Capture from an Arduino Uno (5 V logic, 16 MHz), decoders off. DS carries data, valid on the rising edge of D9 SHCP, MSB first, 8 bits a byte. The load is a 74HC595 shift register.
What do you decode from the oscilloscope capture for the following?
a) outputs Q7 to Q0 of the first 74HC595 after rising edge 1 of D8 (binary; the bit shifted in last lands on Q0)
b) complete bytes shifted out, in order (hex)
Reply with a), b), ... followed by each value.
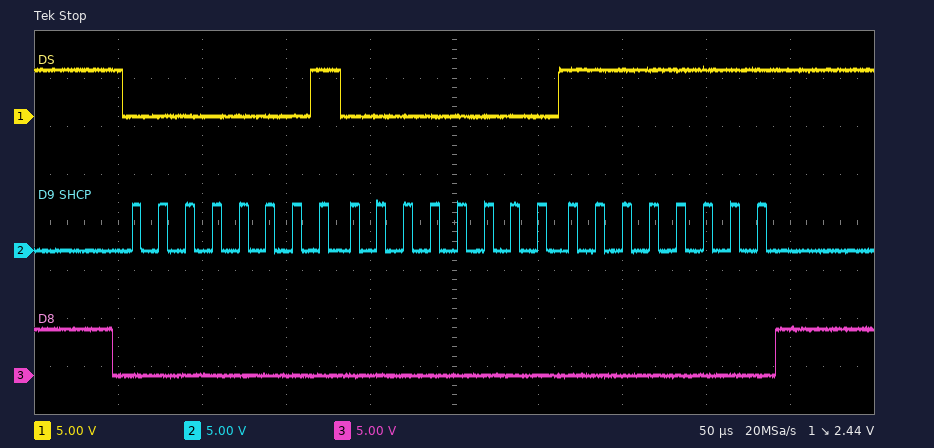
a) 11111111
b) 01 00 FF
